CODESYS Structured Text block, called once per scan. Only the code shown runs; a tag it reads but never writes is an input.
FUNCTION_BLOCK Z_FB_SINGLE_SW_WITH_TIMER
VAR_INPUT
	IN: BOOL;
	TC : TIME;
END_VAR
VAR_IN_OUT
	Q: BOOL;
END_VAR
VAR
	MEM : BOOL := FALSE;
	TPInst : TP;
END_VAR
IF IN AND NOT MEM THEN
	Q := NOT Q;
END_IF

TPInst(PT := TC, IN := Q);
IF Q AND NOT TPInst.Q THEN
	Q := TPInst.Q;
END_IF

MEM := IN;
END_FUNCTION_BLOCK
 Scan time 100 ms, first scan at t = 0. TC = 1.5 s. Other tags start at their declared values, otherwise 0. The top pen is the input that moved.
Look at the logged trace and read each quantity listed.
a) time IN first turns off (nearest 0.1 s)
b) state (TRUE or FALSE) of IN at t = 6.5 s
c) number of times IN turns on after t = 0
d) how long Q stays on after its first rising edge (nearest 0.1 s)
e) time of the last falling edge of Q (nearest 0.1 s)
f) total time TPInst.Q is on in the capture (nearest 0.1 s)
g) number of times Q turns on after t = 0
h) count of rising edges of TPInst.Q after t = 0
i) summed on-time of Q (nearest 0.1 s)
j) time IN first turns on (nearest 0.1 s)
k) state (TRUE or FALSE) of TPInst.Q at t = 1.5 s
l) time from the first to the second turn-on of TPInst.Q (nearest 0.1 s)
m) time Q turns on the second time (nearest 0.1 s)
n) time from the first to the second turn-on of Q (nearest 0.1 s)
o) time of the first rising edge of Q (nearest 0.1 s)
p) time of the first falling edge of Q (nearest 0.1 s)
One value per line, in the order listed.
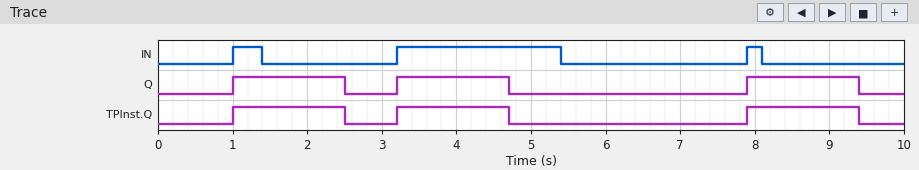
1.4 s
FALSE
3
1.5 s
9.4 s
4.5 s
3
3
4.5 s
1.0 s
TRUE
2.2 s
3.2 s
2.2 s
1.0 s
2.5 s
